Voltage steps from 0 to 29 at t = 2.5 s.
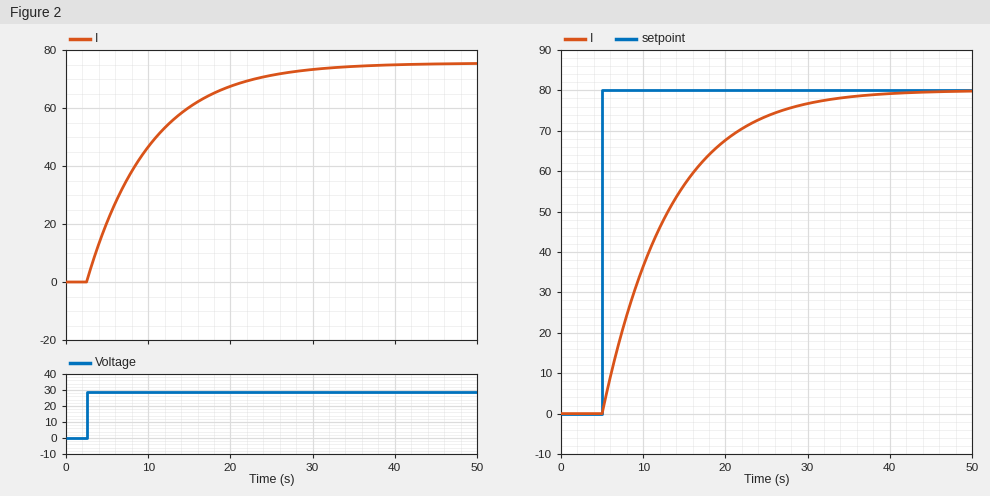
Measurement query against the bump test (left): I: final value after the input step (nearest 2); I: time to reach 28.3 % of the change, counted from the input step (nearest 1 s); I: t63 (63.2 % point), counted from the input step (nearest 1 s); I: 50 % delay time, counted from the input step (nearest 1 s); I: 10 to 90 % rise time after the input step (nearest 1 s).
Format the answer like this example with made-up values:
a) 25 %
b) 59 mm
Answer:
a) 76
b) 3 s
c) 8 s
d) 5 s
e) 17 s
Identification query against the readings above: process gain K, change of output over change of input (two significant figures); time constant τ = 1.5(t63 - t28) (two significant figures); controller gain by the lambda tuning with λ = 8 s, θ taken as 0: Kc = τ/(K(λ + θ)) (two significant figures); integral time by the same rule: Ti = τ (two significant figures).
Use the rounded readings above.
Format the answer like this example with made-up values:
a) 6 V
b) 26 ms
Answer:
a) 2.6
b) 7.5 s
c) 0.36
d) 7.5 s
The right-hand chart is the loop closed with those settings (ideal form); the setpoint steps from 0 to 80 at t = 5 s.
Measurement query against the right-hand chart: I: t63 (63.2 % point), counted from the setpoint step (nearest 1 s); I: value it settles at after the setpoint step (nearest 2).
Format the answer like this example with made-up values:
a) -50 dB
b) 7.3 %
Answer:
a) 8 s
b) 80
